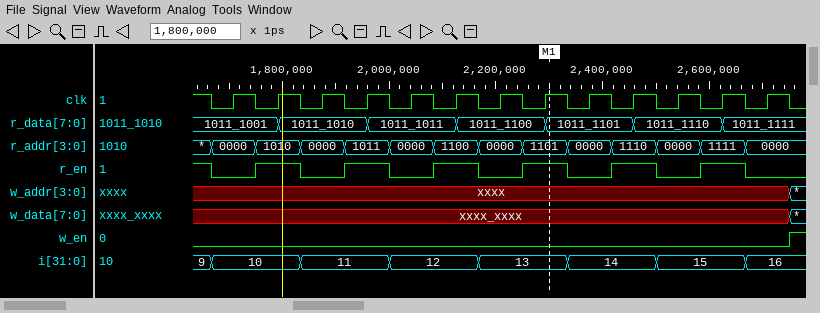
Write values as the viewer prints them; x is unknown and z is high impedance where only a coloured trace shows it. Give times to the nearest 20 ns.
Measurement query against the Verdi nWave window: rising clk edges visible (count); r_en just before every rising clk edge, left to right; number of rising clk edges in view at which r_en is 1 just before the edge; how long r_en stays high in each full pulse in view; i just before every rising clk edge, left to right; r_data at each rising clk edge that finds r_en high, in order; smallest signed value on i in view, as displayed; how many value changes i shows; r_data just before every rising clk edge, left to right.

13
0 1 0 1 0 1 0 1 0 1 0 1 0
6
80 ns, 80 ns, 80 ns, 80 ns, 80 ns, 80 ns
10, 10, 11, 11, 12, 12, 13, 13, 14, 14, 15, 15, 16
1011_1001, 1011_1010, 1011_1011, 1011_1100, 1011_1101, 1011_1110
9
7
1011_1001, 1011_1001, 1011_1010, 1011_1010, 1011_1011, 1011_1011, 1011_1100, 1011_1100, 1011_1101, 1011_1101, 1011_1110, 1011_1110, 1011_1111
